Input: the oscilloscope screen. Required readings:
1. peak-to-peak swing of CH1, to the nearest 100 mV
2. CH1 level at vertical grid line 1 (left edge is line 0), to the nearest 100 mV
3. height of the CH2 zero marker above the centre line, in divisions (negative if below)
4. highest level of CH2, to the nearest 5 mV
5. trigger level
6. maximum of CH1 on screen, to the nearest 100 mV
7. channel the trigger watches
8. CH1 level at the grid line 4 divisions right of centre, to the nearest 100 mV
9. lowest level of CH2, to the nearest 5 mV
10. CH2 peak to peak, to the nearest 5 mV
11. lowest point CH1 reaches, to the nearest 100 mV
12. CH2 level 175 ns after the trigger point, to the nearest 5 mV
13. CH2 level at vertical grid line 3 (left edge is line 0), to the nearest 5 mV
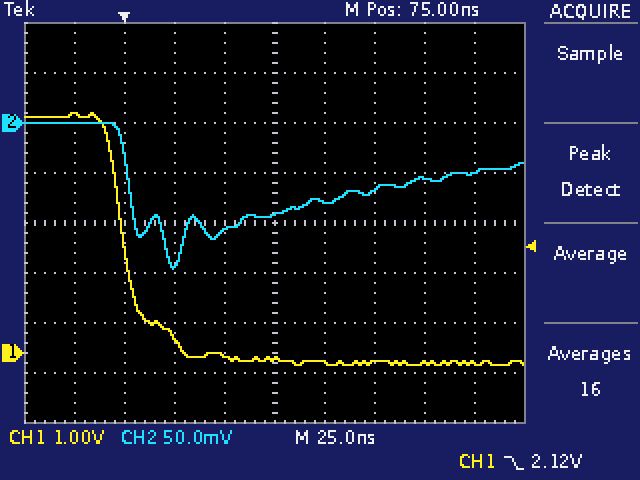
5.0 V
4.8 V
+2.0 div
0 mV
2.12 V
4.8 V
CH1
-200 mV
-145 mV
145 mV
-200 mV
-50 mV
-140 mV
